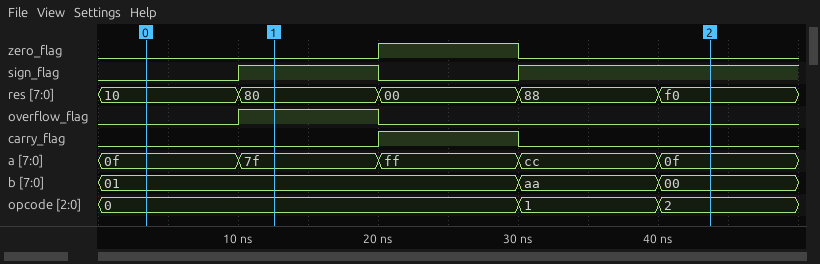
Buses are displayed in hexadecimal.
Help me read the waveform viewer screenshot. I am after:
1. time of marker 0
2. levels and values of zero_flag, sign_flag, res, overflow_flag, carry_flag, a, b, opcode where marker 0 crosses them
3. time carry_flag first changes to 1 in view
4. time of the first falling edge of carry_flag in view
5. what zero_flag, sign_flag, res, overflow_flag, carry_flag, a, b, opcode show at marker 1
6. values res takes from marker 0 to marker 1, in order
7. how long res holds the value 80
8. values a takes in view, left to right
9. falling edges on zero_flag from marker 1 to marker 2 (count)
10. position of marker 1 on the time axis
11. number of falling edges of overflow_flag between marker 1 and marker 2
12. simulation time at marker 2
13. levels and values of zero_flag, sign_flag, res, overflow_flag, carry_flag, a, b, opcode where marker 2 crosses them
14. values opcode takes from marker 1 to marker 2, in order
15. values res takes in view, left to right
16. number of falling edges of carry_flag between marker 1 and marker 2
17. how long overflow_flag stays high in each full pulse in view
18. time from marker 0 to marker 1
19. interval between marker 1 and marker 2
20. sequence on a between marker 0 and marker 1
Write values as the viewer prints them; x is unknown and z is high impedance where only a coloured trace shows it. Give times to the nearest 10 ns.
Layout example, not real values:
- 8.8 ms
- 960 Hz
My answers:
- 0 ns
- zero_flag=0, sign_flag=0, res=10, overflow_flag=0, carry_flag=0, a=0f, b=01, opcode=0
- 20 ns
- 30 ns
- zero_flag=0, sign_flag=1, res=80, overflow_flag=1, carry_flag=0, a=7f, b=01, opcode=0
- 10, 80
- 10 ns
- 0f, 7f, ff, cc, 0f
- 1
- 10 ns
- 1
- 40 ns
- zero_flag=0, sign_flag=1, res=f0, overflow_flag=0, carry_flag=0, a=0f, b=00, opcode=2
- 0, 1, 2
- 10, 80, 00, 88, f0
- 1
- 10 ns
- 10 ns
- 30 ns
- 0f, 7f
